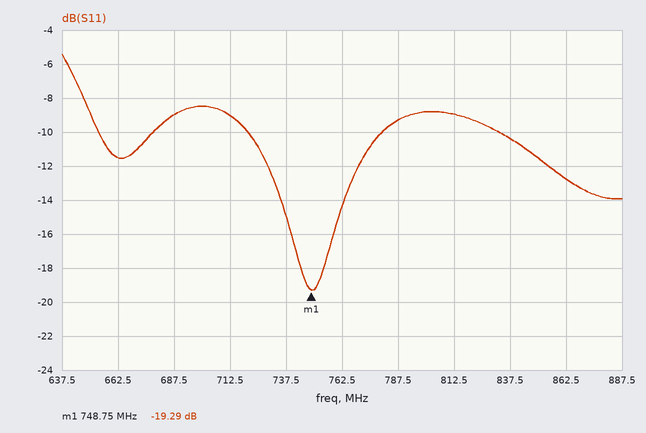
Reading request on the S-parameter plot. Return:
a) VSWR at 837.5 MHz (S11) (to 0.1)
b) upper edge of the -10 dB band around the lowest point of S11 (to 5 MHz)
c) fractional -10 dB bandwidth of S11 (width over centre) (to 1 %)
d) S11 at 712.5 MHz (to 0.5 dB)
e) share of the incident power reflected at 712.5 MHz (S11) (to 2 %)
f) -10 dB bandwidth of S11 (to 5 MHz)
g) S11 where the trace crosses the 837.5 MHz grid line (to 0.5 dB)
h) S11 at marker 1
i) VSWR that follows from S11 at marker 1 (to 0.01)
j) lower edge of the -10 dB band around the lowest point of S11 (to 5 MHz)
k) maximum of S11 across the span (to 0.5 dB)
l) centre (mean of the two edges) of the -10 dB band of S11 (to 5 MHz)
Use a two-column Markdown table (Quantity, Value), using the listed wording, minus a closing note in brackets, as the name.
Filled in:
| Quantity | Value |
|---|---|
| VSWR at 837.5 MHz (S11) | 1.9 |
| upper edge of the -10 dB band around the lowest point of S11 | 780 MHz |
| fractional -10 dB bandwidth of S11 (width over centre) | 8 % |
| S11 at 712.5 MHz | -9.0 dB |
| share of the incident power reflected at 712.5 MHz (S11) | 12 % |
| -10 dB bandwidth of S11 | 60 MHz |
| S11 where the trace crosses the 837.5 MHz grid line | -10.5 dB |
| S11 at marker 1 | -19.29 dB |
| VSWR that follows from S11 at marker 1 | 1.24 |
| lower edge of the -10 dB band around the lowest point of S11 | 720 MHz |
| maximum of S11 across the span | -5.5 dB |
| centre (mean of the two edges) of the -10 dB band of S11 | 750 MHz |
